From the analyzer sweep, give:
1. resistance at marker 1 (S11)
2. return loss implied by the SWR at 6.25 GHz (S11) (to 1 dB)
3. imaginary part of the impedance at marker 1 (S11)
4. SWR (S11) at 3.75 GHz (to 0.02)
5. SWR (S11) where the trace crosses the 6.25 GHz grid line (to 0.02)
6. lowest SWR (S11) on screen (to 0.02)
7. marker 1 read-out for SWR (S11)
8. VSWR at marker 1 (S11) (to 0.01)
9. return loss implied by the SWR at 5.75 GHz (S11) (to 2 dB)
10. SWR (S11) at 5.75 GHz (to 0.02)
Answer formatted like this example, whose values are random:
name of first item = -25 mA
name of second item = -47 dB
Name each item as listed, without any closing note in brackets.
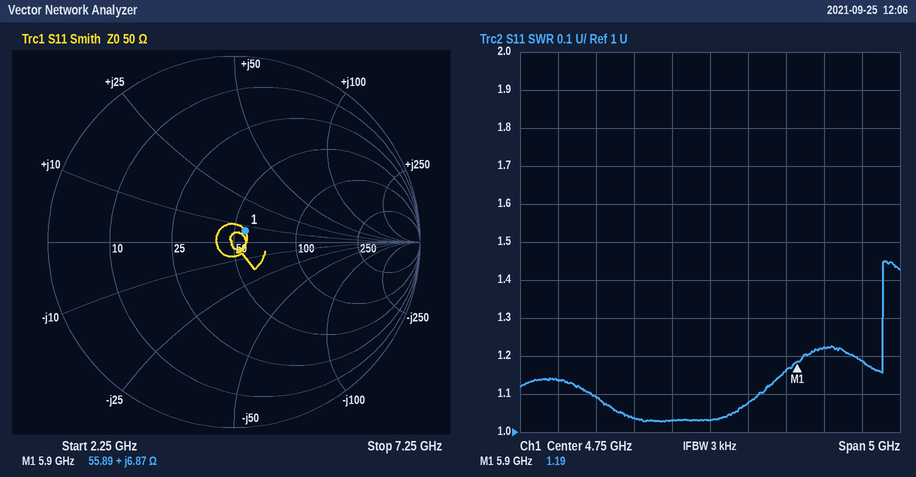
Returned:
resistance at marker 1 = 55.89 Ω
return loss implied by the SWR at 6.25 GHz (S11) = 20 dB
imaginary part of the impedance at marker 1 = +6.87 Ω
SWR (S11) at 3.75 GHz = 1.04
SWR (S11) where the trace crosses the 6.25 GHz grid line = 1.22
lowest SWR (S11) on screen = 1.02
marker 1 read-out for SWR = 1.19
VSWR at marker 1 (S11) = 1.19
return loss implied by the SWR at 5.75 GHz (S11) = 22 dB
SWR (S11) at 5.75 GHz = 1.16
